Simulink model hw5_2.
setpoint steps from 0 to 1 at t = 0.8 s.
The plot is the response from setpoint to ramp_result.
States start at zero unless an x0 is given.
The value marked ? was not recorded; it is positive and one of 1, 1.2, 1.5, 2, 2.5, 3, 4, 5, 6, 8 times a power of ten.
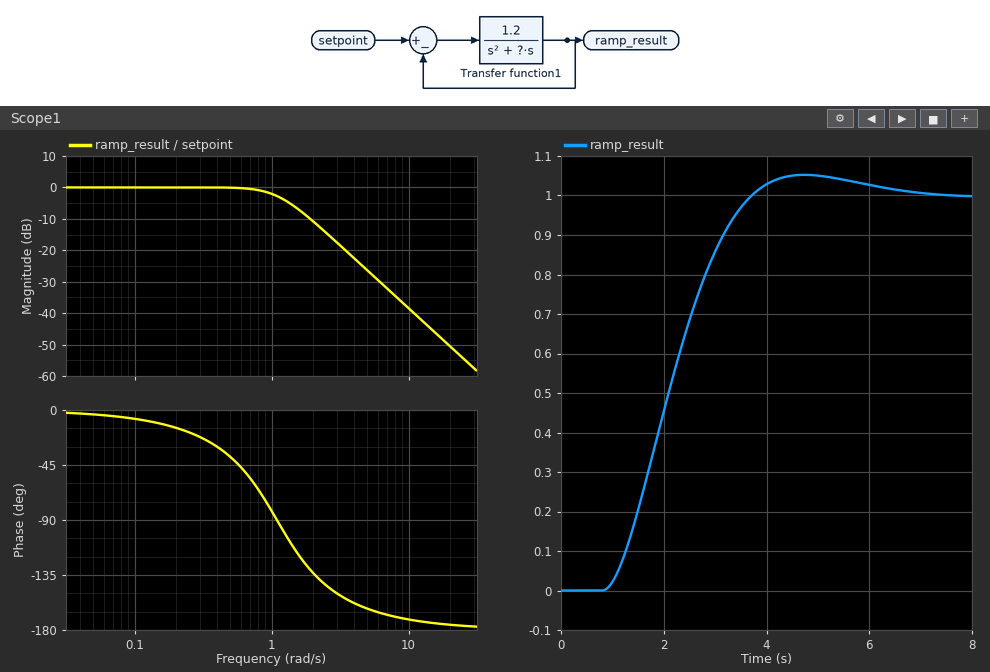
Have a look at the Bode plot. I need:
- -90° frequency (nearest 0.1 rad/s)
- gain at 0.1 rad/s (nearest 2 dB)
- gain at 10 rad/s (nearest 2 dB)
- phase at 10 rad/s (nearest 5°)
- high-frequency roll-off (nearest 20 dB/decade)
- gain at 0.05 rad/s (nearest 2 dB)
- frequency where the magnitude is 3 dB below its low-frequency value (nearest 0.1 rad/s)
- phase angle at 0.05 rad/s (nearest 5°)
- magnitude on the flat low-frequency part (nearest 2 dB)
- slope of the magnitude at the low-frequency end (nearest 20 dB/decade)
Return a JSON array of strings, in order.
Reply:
["1.1 rad/s", "0 dB", "-38 dB", "-170°", "-40 dB/decade", "0 dB", "1.1 rad/s", "-5°", "0 dB", "0 dB/decade"]
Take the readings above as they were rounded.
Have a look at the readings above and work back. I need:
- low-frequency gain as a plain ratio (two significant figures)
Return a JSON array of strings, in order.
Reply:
["1.0"]
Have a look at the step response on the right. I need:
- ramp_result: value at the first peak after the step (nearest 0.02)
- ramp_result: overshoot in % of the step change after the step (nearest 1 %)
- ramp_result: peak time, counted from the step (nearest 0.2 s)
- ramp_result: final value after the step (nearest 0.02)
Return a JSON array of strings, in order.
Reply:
["1.06", "5 %", "4.0 s", "1.00"]
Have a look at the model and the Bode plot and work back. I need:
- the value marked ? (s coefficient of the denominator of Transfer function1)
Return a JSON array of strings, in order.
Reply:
["1.5"]
